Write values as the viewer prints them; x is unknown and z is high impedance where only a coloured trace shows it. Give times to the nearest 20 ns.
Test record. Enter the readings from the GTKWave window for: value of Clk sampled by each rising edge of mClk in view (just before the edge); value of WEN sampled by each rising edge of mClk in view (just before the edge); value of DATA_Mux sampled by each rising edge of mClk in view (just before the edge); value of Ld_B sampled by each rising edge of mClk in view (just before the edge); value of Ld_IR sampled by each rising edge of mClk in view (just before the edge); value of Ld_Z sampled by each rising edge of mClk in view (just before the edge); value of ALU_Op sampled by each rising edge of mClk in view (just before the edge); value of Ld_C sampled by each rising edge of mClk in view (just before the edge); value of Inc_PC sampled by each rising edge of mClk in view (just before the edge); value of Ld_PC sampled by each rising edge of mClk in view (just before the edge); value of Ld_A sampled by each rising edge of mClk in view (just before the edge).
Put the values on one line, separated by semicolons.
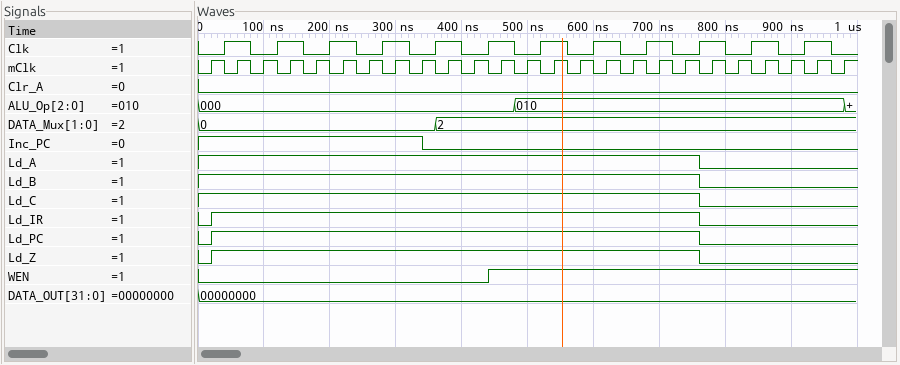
0 1 0 1 0 1 0 1 0 1 0 1 0 1 0 1 0 1 0 1 0 1 0 1 0; 0 0 0 0 0 0 0 0 0 0 0 1 1 1 1 1 1 1 1 1 1 1 1 1 1; 0, 0, 0, 0, 0, 0, 0, 0, 0, 2, 2, 2, 2, 2, 2, 2, 2, 2, 2, 2, 2, 2, 2, 2, 2; 1 1 1 1 1 1 1 1 1 1 1 1 1 1 1 1 1 1 1 0 0 0 0 0 0; 0 1 1 1 1 1 1 1 1 1 1 1 1 1 1 1 1 1 1 0 0 0 0 0 0; 0 1 1 1 1 1 1 1 1 1 1 1 1 1 1 1 1 1 1 0 0 0 0 0 0; 000, 000, 000, 000, 000, 000, 000, 000, 000, 000, 000, 000, 010, 010, 010, 010, 010, 010, 010, 010, 010, 010, 010, 010, 010; 1 1 1 1 1 1 1 1 1 1 1 1 1 1 1 1 1 1 1 0 0 0 0 0 0; 1 1 1 1 1 1 1 1 1 0 0 0 0 0 0 0 0 0 0 0 0 0 0 0 0; 0 1 1 1 1 1 1 1 1 1 1 1 1 1 1 1 1 1 1 0 0 0 0 0 0; 1 1 1 1 1 1 1 1 1 1 1 1 1 1 1 1 1 1 1 0 0 0 0 0 0
